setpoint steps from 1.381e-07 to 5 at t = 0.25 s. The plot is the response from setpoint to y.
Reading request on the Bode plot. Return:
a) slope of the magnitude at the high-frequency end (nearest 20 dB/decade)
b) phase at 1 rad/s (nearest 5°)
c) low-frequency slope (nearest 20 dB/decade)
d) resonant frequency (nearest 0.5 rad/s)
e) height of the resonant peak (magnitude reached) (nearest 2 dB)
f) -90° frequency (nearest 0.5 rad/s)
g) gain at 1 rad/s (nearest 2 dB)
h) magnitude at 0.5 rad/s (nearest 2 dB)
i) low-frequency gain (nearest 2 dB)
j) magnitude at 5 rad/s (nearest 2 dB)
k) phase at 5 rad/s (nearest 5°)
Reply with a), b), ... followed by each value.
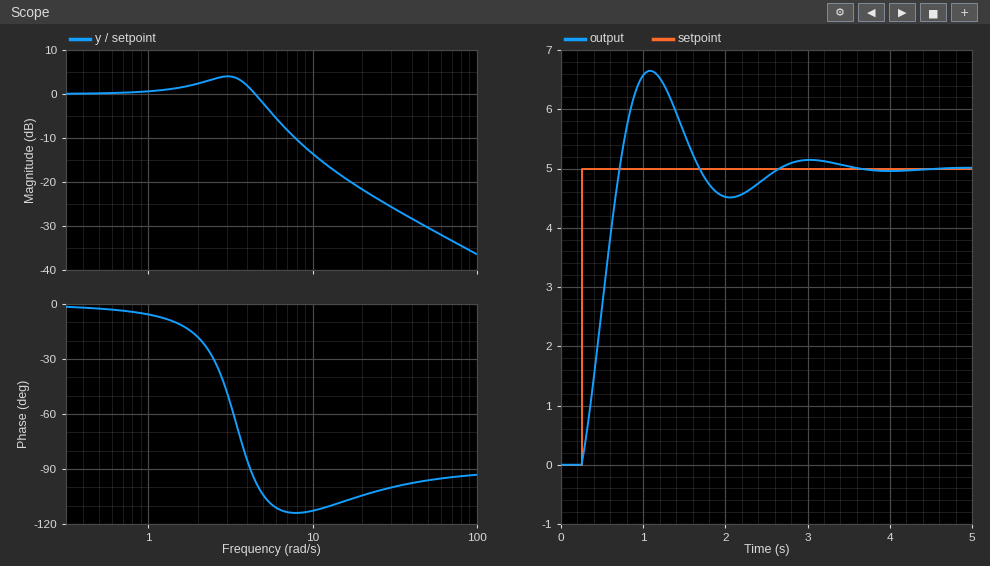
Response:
a) -20 dB/decade
b) -5°
c) 0 dB/decade
d) 3.0 rad/s
e) 4 dB
f) 4.0 rad/s
g) 0 dB
h) 0 dB
i) 0 dB
j) -2 dB
k) -105°
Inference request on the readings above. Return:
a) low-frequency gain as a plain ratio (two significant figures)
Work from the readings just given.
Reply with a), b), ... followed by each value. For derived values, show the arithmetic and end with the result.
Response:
a) 10^(0 / 20) = 1.0
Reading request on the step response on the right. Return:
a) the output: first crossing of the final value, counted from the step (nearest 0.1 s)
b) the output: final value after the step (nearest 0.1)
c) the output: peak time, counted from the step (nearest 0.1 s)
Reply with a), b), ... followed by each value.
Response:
a) 0.5 s
b) 5.0
c) 0.8 s
